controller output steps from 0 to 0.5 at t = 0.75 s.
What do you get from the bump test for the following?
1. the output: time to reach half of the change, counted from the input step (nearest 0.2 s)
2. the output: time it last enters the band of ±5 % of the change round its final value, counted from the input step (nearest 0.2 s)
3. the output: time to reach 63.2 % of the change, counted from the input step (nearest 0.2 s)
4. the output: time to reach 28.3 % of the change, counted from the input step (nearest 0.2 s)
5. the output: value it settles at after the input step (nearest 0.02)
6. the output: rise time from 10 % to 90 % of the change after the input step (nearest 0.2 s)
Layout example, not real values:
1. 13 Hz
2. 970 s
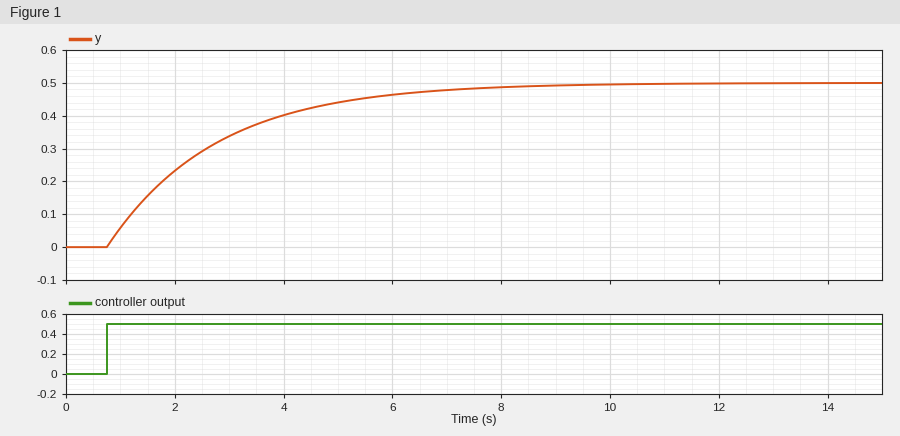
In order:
1. 1.4 s
2. 6.0 s
3. 2.0 s
4. 0.6 s
5. 0.50
6. 4.4 s
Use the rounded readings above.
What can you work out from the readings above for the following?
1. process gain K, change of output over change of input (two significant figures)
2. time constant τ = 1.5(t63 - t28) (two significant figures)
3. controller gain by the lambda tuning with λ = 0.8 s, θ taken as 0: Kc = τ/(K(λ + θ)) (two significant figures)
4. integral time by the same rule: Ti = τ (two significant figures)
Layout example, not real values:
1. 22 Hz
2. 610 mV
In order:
1. 1.0
2. 2.1 s
3. 2.6
4. 2.1 s
